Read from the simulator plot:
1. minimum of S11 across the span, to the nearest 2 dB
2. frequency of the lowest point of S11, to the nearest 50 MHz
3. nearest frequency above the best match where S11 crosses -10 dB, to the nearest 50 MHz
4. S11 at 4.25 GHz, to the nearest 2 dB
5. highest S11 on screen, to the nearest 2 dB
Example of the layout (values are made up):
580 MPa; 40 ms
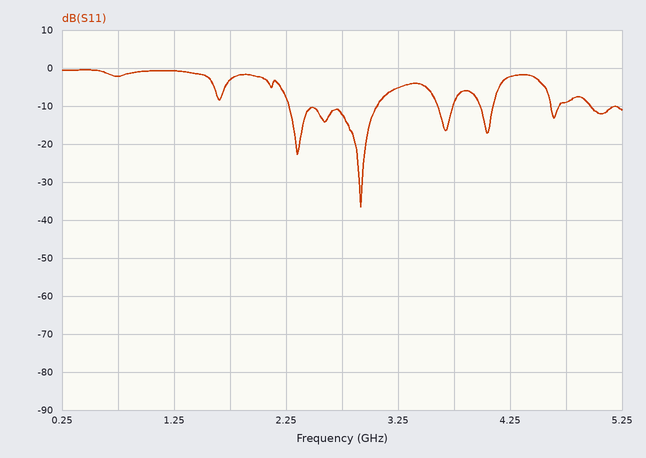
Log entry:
-36 dB; 2.90 GHz; 3.05 GHz; -2 dB; 0 dB
